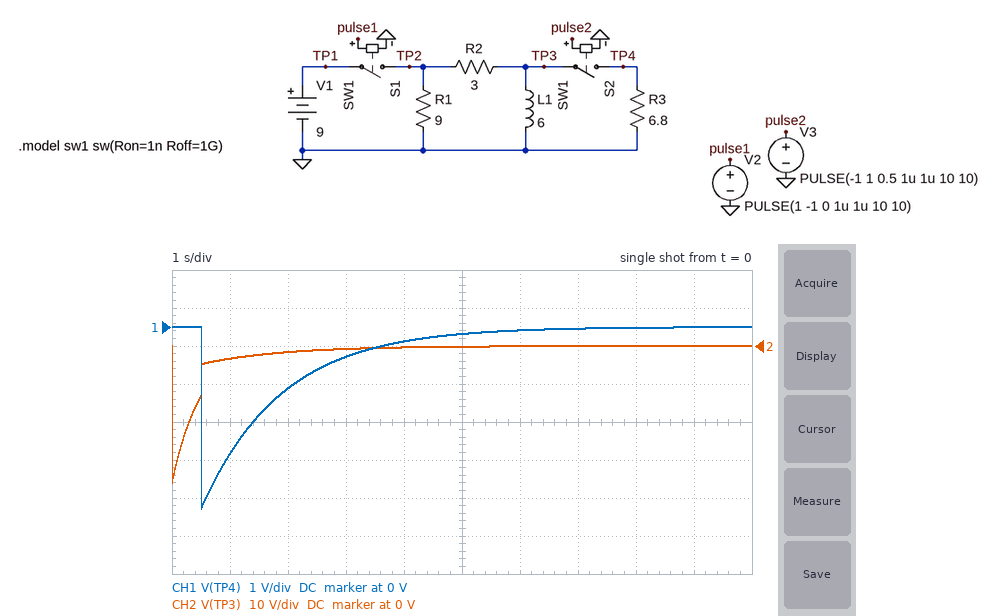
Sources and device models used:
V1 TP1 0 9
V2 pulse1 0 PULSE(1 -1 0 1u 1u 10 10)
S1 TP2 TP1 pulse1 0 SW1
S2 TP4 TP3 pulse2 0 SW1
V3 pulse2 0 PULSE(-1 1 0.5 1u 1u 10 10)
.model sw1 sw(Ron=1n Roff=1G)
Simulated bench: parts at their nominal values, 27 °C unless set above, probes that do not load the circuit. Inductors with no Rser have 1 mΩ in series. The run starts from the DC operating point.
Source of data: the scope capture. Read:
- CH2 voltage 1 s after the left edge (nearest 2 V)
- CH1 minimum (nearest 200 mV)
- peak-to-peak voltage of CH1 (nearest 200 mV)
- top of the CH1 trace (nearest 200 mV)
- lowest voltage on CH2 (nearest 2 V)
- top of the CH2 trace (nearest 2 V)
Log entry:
-4 V
-4.8 V
4.8 V
0 V
-36 V
0 V
